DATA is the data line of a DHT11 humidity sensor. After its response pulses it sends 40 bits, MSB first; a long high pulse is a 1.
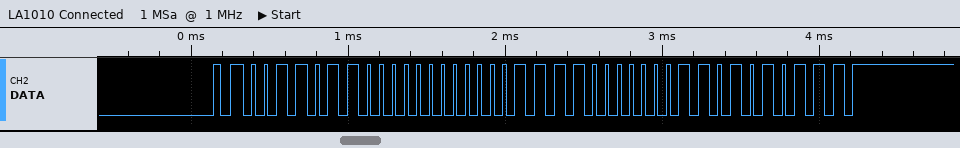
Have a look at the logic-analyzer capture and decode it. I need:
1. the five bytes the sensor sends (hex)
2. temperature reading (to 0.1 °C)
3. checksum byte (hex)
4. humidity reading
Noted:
36 00 1E 03 57
30.3 °C
0x57
54 %
